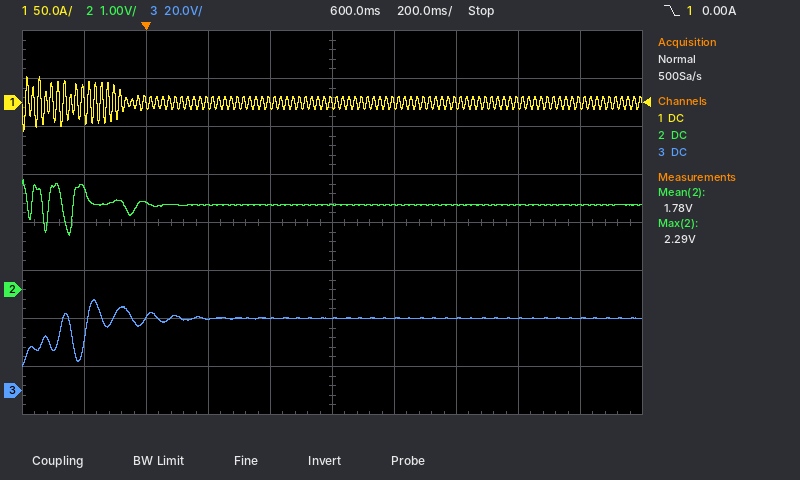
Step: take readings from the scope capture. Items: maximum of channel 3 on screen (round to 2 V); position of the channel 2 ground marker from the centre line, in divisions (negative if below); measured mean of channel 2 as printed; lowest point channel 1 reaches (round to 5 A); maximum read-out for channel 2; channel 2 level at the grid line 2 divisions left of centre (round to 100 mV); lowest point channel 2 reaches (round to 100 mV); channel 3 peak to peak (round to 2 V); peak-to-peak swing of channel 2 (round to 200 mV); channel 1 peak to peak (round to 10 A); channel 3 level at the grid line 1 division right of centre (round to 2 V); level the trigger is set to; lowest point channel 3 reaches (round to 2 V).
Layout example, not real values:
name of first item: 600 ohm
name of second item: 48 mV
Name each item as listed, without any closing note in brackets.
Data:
maximum of channel 3 on screen: 38 V
position of the channel 2 ground marker from the centre line, in divisions: -1.4 div
measured mean of channel 2 as printed: 1.78 V
lowest point channel 1 reaches: -30 A
maximum read-out for channel 2: 2.29 V
channel 2 level at the grid line 2 divisions left of centre: 1.8 V
lowest point channel 2 reaches: 1.1 V
channel 3 peak to peak: 28 V
peak-to-peak swing of channel 2: 1.2 V
channel 1 peak to peak: 60 A
channel 3 level at the grid line 1 division right of centre: 30 V
level the trigger is set to: 0.00 A
lowest point channel 3 reaches: 10 V
